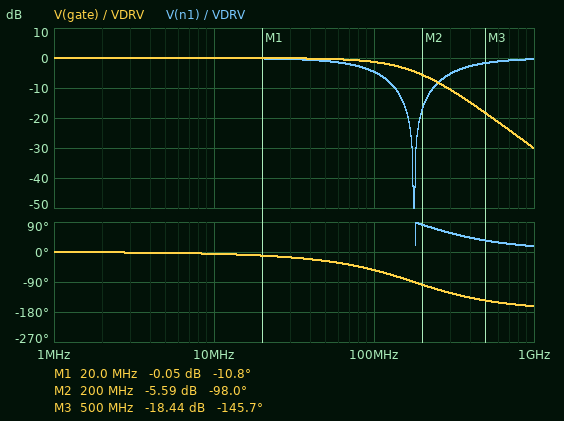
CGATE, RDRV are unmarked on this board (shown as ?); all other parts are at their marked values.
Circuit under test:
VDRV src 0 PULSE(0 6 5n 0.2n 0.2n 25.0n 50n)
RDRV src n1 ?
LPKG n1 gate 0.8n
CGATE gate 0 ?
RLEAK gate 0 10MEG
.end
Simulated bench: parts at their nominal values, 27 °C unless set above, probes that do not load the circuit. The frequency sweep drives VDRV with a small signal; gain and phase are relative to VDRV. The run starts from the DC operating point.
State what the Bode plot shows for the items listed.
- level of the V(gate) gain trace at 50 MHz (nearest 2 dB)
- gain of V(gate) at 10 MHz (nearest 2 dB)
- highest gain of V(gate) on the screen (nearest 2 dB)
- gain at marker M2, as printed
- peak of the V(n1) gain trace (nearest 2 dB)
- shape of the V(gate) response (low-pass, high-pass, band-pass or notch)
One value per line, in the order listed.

0 dB
0 dB
0 dB
-5.59 dB
0 dB
low-pass
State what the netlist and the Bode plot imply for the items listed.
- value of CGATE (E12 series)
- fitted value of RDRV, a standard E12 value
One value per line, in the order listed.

1 nF
1.5 Ω
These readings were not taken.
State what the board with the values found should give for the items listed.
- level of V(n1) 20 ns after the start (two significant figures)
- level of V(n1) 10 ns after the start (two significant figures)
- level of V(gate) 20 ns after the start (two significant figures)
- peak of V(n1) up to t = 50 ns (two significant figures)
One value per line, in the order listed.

6.0 V
6.0 V
6.0 V
6.0 V
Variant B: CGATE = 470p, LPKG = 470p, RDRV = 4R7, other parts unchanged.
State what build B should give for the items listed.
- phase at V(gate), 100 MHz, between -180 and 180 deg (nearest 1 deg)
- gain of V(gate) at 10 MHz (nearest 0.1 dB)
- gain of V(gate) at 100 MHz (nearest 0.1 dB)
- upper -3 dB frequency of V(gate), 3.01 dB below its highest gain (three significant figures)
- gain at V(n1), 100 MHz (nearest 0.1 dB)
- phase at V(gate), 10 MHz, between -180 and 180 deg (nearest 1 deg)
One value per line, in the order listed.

-57 deg
-0.1 dB
-4.4 dB
75.5 MHz
-5.2 dB
-8 deg
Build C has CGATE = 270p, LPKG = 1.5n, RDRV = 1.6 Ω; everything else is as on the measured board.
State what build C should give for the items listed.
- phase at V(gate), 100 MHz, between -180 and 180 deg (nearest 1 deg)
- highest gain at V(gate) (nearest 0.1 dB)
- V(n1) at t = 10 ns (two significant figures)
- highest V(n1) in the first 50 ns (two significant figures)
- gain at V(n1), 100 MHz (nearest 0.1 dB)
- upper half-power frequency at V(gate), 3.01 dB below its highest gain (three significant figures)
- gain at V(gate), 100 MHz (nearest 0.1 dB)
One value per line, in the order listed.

-18 deg
3.9 dB
5.7 V
6.8 V
-0.4 dB
297 MHz
1.1 dB
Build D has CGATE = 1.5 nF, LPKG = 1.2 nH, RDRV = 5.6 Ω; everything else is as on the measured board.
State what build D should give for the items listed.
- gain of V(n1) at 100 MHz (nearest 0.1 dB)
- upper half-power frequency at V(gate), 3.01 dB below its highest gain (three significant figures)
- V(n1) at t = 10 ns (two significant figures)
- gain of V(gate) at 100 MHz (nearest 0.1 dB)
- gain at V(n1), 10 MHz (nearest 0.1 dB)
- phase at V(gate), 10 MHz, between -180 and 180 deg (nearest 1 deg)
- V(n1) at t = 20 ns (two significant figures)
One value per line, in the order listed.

-25.2 dB
19.4 MHz
2.5 V
-14.5 dB
-1.1 dB
-28 deg
5.0 V
